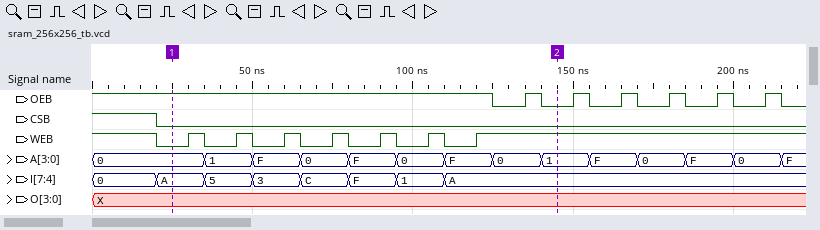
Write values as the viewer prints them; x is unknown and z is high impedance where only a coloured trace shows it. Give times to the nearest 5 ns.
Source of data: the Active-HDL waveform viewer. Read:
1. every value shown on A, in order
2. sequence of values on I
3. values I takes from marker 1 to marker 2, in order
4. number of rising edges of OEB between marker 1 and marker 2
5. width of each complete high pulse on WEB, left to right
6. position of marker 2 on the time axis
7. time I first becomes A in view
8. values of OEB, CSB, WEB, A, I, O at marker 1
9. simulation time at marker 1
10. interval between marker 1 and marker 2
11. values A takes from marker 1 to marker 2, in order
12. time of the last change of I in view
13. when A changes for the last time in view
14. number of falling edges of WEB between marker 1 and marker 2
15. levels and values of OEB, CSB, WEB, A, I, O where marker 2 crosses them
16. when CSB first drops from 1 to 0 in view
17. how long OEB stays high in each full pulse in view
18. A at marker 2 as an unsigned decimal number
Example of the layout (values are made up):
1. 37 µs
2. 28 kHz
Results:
1. 0, 1, F, 0, F, 0, F, 0, 1, F, 0, F, 0, F
2. 0, A, 5, 3, C, F, 1, A
3. A, 5, 3, C, F, 1, A
4. 1
5. 5 ns, 5 ns, 5 ns, 5 ns, 5 ns, 5 ns
6. 145 ns
7. 20 ns
8. OEB=1, CSB=0, WEB=0, A=0, I=A, O=X
9. 25 ns
10. 120 ns
11. 0, 1, F, 0, F, 0, F, 0, 1
12. 110 ns
13. 215 ns
14. 6
15. OEB=0, CSB=0, WEB=1, A=1, I=A, O=X
16. 20 ns
17. 5 ns, 5 ns, 5 ns, 5 ns, 5 ns, 5 ns
18. 1
